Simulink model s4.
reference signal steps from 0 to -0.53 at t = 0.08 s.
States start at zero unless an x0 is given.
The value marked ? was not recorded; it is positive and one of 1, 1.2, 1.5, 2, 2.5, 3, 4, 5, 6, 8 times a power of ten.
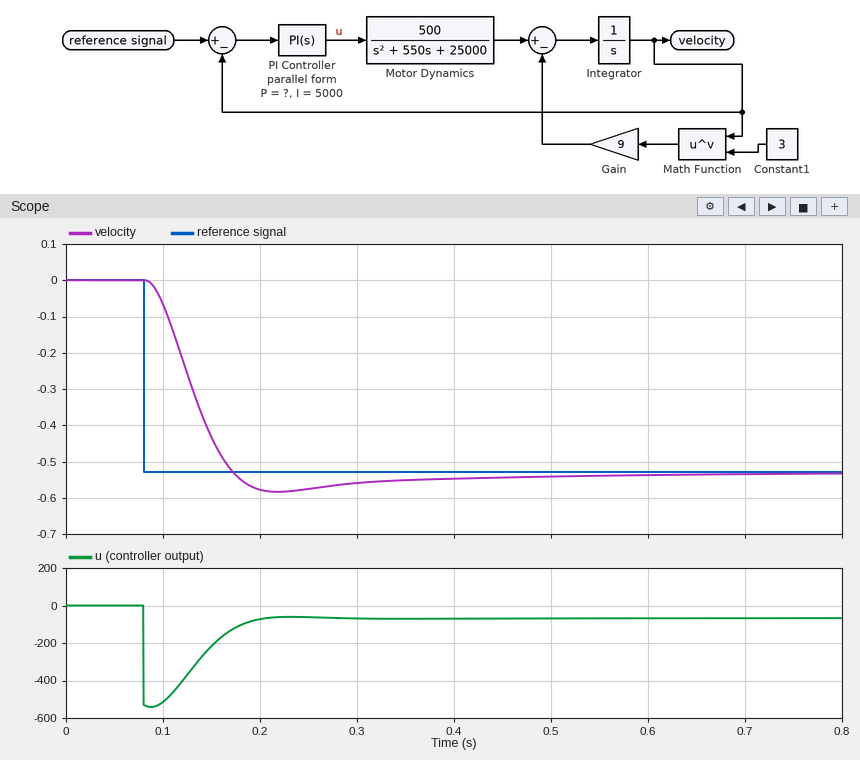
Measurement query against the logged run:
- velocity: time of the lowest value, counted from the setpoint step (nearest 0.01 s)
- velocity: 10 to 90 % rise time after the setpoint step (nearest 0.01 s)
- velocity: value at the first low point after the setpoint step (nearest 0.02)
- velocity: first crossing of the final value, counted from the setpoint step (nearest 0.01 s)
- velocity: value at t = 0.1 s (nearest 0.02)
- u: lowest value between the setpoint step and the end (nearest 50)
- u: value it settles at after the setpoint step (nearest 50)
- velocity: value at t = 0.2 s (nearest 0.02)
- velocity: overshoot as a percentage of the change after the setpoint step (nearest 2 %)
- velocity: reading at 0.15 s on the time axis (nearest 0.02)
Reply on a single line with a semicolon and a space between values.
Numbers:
0.14 s; 0.06 s; -0.58; 0.09 s; -0.06; -550; -50; -0.58; 10 %; -0.44
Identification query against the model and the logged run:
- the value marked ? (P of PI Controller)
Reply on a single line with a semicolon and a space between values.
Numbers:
1000
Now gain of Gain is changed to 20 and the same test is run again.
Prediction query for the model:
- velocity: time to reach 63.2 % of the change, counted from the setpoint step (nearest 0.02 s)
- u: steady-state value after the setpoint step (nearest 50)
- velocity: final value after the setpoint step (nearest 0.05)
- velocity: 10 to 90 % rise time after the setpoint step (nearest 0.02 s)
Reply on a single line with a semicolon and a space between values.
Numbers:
0.06 s; -150; -0.55; 0.06 s
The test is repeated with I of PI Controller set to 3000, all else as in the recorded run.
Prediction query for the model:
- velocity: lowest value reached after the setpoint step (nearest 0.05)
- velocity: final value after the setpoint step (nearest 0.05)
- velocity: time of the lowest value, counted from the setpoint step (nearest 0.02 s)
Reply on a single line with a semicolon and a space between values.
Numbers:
-0.55; -0.55; 0.14 s
